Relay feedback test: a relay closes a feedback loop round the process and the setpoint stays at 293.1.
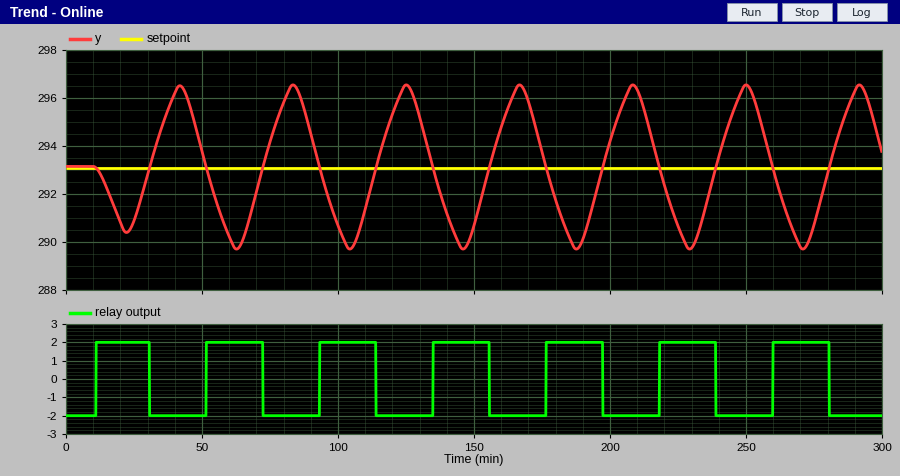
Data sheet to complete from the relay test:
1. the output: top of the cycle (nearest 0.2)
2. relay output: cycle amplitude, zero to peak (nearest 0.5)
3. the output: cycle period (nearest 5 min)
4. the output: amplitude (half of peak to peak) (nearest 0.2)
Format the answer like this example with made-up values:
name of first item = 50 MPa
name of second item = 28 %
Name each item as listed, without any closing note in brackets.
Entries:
the output: top of the cycle = 296.6
relay output: cycle amplitude, zero to peak = 2.0
the output: cycle period = 40 min
the output: amplitude (half of peak to peak) = 3.4
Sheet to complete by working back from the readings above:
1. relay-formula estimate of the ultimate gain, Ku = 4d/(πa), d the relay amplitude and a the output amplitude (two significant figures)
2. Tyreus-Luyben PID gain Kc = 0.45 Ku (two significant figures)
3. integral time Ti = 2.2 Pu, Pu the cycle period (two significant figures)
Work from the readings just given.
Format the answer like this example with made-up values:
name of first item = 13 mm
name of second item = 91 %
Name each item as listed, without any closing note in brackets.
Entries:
relay-formula estimate of the ultimate gain, Ku = 4d/(πa), d the relay amplitude and a the output amplitude = 0.75
Tyreus-Luyben PID gain Kc = 0.45 Ku = 0.34
integral time Ti = 2.2 Pu, Pu the cycle period = 88 min
